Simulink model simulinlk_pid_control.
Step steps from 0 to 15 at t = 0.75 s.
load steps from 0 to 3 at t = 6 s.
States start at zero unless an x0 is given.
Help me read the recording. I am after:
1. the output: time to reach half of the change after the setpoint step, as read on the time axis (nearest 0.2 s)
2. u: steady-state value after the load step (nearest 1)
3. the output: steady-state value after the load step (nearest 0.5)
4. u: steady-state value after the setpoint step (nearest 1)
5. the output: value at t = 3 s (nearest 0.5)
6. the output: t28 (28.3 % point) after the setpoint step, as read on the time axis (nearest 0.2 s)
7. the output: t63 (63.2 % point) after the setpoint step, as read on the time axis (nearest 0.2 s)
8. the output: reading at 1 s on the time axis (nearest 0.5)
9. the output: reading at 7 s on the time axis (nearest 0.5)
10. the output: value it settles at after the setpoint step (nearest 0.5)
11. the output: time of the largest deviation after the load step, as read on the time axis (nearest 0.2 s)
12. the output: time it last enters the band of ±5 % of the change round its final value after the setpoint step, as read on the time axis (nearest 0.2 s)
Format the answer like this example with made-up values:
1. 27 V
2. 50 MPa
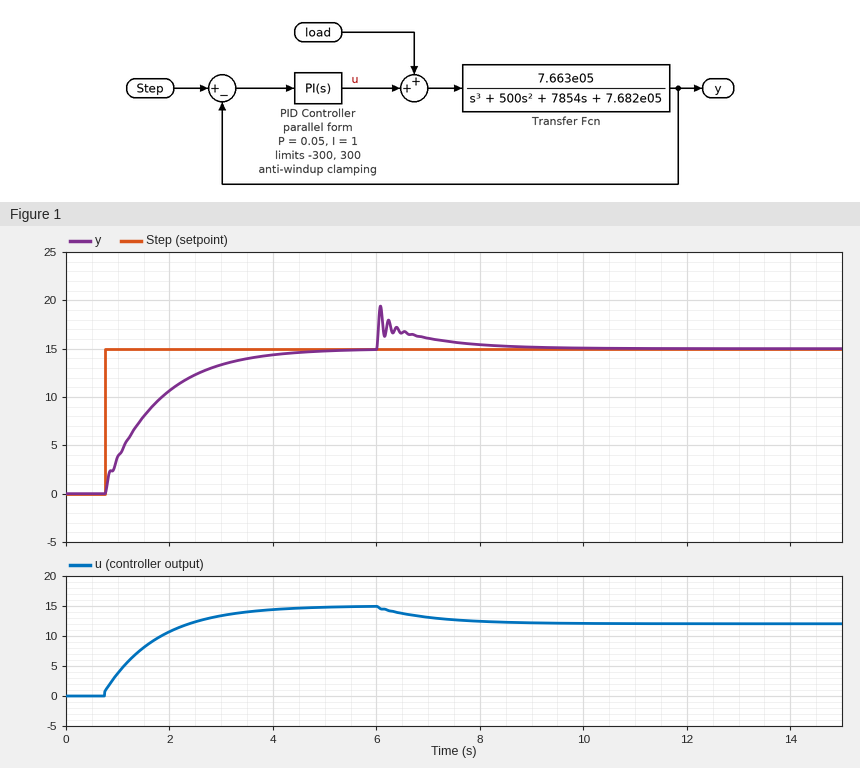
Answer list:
1. 1.4 s
2. 12
3. 15.0
4. 15
5. 13.5
6. 1.0 s
7. 1.8 s
8. 4.0
9. 16.0
10. 15.0
11. 6.0 s
12. 3.8 s
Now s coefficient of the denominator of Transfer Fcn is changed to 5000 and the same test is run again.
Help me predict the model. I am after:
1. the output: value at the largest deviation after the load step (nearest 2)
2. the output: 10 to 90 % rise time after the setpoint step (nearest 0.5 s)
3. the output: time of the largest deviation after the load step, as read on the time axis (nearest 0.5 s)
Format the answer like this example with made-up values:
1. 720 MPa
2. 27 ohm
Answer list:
1. 20
2. 2.5 s
3. 6.0 s
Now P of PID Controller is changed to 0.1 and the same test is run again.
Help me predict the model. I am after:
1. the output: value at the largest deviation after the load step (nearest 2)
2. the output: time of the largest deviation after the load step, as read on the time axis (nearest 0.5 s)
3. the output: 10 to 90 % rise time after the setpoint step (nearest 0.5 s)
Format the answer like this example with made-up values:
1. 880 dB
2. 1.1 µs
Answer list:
1. 20
2. 6.0 s
3. 2.5 s
